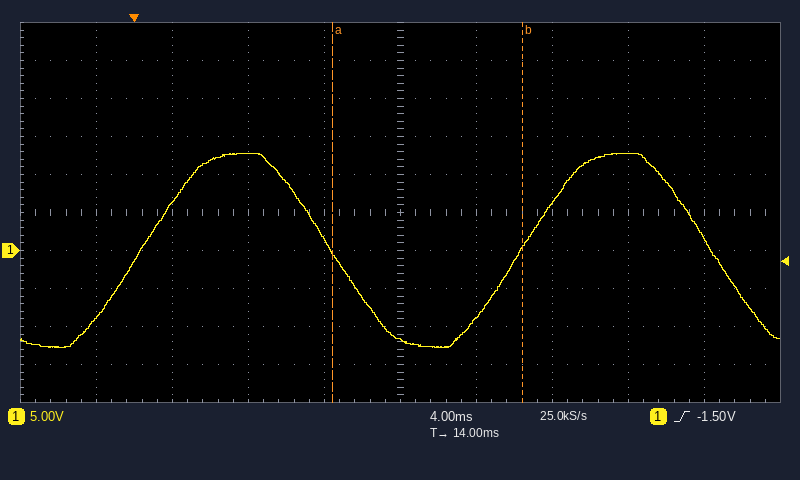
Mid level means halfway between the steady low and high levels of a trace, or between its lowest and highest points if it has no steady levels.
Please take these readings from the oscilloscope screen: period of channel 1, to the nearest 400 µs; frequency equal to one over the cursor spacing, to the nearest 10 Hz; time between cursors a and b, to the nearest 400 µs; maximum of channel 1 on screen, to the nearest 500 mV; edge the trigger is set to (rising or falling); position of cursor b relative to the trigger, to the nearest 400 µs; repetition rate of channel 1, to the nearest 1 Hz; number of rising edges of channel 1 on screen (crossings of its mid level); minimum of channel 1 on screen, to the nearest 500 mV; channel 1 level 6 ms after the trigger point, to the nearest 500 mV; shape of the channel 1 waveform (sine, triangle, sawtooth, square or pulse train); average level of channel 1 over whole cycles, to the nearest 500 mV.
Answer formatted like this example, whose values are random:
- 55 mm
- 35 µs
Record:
- 20.0 ms
- 100 Hz
- 10.0 ms
- 13.0 V
- rising
- +20.4 ms
- 50 Hz
- 2
- -13.0 V
- 13.0 V
- sine
- 0.0 V
